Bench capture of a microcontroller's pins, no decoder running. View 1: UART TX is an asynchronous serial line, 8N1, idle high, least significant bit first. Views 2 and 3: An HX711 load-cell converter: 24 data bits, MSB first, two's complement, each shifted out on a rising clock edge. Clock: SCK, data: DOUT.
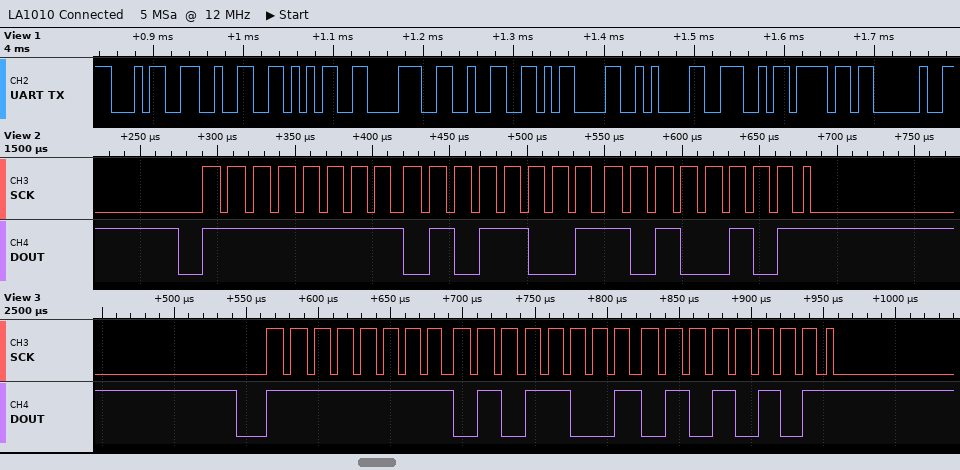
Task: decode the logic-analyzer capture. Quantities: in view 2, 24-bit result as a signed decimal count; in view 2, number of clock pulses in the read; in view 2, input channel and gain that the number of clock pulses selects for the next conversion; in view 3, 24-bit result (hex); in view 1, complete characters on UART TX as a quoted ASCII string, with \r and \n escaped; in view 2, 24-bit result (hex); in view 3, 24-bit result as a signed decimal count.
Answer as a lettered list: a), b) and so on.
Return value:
a) -42587
b) 25
c) channel A, gain 128
d) 0xFF5955
e) "42582\r\nNo "
f) 0xFF59A5
g) -42667
